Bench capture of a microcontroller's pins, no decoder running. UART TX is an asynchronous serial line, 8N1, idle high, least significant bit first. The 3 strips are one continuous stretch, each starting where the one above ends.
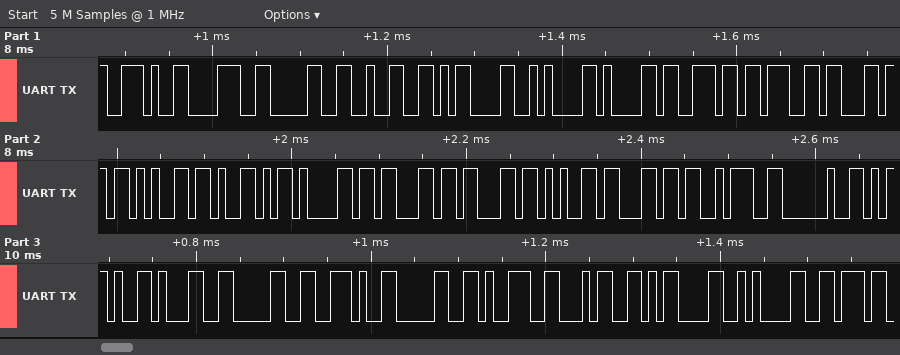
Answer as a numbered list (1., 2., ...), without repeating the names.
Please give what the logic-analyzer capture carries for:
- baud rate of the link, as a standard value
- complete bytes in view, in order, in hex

1. 115200 baud
2. 2E 38 30 32 0D 0A 61 6E 67 6C 65 59 61 63 63 65 6C 3A 20 2D 31 30 2E 30 39 34 0D 0A 76
